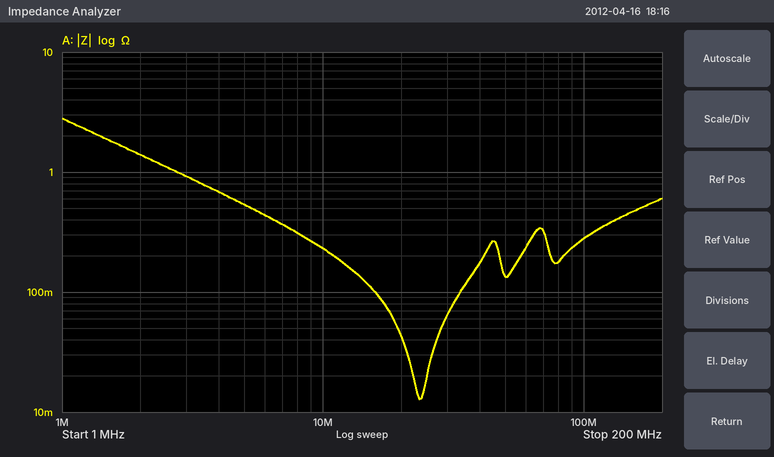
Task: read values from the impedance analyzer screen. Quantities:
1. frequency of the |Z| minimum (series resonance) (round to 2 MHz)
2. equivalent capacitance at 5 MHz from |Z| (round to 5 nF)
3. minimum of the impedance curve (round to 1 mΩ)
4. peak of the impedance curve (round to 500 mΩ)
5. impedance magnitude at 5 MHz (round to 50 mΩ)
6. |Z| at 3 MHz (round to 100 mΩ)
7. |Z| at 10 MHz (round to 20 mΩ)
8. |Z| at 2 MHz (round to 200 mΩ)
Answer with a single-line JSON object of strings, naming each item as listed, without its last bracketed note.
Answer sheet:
{"frequency of the |Z| minimum (series resonance)": "24 MHz", "equivalent capacitance at 5 MHz from |Z|": "60 nF", "minimum of the impedance curve": "13 mΩ", "peak of the impedance curve": "3.0 Ω", "impedance magnitude at 5 MHz": "550 mΩ", "|Z| at 3 MHz": "900 mΩ", "|Z| at 10 MHz": "240 mΩ", "|Z| at 2 MHz": "1.4 Ω"}
